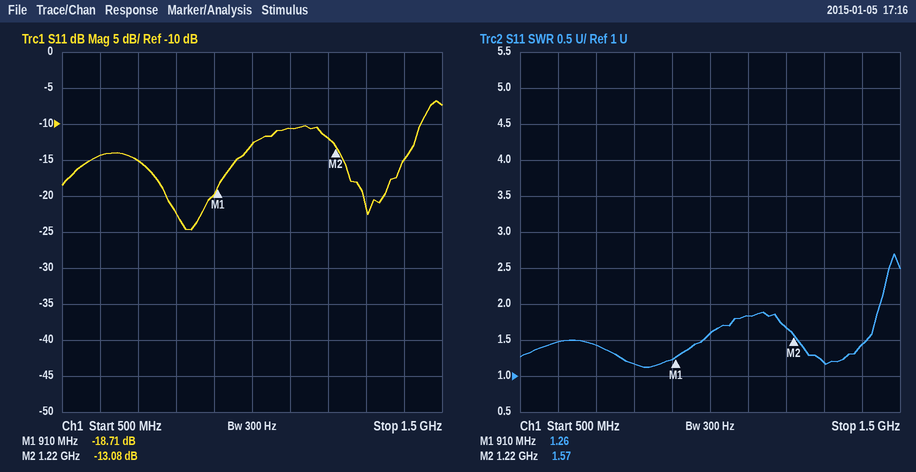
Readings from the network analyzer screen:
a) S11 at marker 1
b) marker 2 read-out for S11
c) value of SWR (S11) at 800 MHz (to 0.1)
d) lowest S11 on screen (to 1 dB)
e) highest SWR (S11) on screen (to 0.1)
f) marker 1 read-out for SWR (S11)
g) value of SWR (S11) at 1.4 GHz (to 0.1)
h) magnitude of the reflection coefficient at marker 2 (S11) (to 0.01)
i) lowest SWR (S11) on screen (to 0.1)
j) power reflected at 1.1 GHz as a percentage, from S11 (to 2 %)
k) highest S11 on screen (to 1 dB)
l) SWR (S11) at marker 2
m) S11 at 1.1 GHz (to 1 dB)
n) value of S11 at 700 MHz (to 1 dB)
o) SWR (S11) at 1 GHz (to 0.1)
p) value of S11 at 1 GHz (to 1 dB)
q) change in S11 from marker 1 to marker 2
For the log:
-18.71 dB
-13.08 dB
1.2
-25 dB
2.7
1.26
1.4
0.22
1.1
8 %
-7 dB
1.57
-11 dB
-15 dB
1.6
-13 dB
5.63 dB
